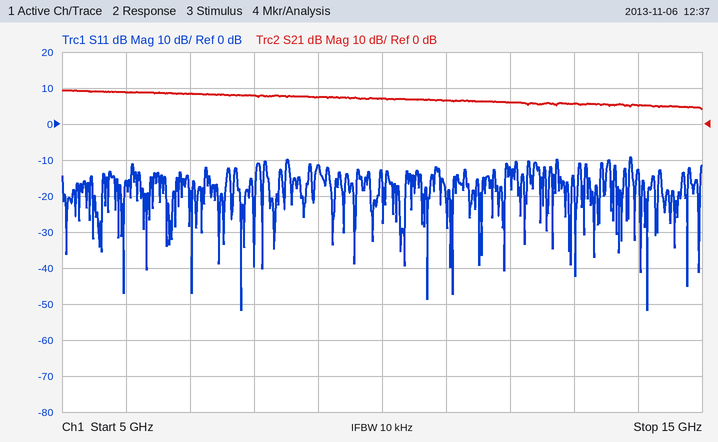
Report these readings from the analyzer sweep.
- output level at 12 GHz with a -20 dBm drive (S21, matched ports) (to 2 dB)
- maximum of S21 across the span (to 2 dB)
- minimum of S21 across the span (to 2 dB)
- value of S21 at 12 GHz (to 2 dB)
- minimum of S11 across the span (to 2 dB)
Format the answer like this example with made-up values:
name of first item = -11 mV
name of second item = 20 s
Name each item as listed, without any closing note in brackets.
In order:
output level at 12 GHz with a -20 dBm drive (S21, matched ports) = -14 dBm
maximum of S21 across the span = 10 dB
minimum of S21 across the span = 4 dB
value of S21 at 12 GHz = 6 dB
minimum of S11 across the span = -52 dB
